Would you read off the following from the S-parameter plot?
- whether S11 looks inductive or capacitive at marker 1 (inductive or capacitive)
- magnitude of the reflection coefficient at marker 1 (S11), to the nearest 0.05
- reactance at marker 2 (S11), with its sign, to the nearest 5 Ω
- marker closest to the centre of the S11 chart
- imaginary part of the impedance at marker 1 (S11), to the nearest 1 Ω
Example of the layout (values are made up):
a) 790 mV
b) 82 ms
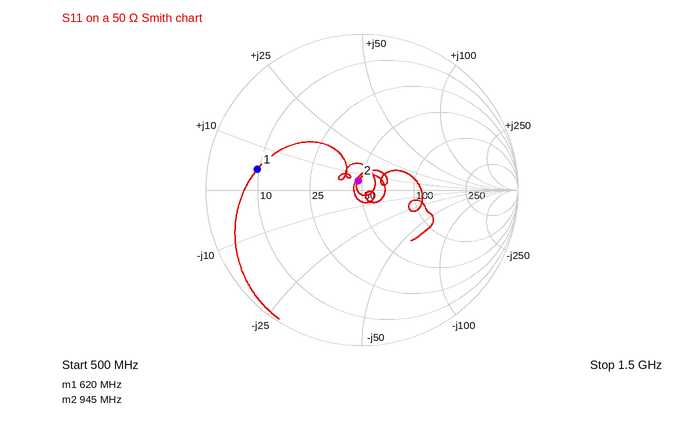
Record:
a) inductive
b) 0.70
c) +5 Ω
d) marker 2
e) +5 Ω
